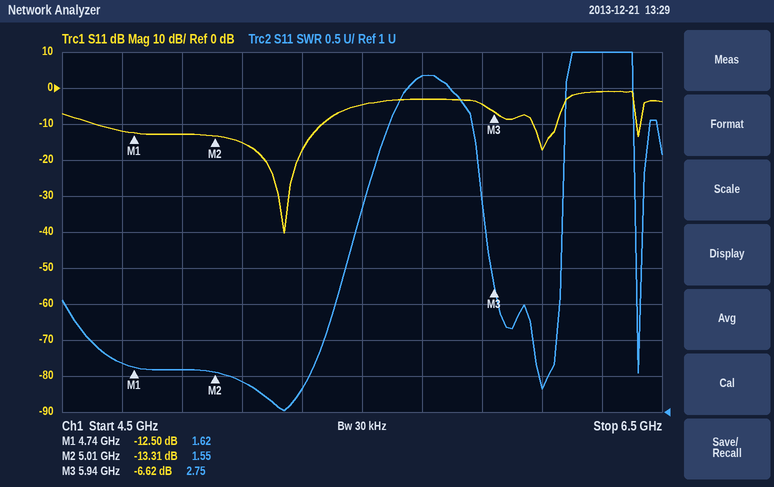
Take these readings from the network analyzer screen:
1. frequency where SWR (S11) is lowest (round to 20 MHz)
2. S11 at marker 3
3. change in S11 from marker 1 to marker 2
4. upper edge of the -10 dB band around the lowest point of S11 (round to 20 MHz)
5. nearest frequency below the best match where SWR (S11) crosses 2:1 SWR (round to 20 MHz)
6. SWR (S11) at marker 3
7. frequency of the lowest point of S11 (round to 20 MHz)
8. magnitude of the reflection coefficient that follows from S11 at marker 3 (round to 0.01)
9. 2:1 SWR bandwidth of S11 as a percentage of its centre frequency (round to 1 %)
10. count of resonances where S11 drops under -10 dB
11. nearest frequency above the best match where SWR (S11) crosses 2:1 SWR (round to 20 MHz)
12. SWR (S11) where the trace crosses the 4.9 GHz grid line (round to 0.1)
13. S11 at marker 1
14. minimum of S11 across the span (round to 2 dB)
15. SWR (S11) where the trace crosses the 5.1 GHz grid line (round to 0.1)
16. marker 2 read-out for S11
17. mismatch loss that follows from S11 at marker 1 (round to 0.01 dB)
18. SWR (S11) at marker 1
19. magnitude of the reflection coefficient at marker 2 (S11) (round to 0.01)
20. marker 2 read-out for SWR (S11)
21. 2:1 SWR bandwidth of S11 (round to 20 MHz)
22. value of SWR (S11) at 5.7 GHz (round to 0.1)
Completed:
5.24 GHz
-6.62 dB
-0.81 dB
5.36 GHz
4.60 GHz
2.75
5.24 GHz
0.47
16 %
3
5.38 GHz
1.6
-12.50 dB
-40 dB
1.4
-13.31 dB
0.25 dB
1.62
0.22
1.55
780 MHz
5.7
